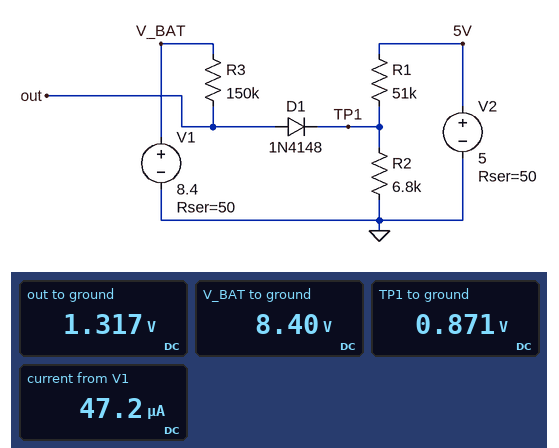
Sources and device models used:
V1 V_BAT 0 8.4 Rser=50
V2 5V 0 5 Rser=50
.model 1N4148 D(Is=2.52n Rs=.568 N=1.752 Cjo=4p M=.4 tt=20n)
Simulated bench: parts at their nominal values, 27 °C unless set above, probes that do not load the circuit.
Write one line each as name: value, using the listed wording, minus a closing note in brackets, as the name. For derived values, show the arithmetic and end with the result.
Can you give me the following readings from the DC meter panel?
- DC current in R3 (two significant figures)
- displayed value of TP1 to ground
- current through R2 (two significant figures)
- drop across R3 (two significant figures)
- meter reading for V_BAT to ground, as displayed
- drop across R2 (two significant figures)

DC current in R3: (8.4 V - 1.317 V) / 150 kΩ = 47 µA
displayed value of TP1 to ground: 0.871 V
current through R2: (871 mV) / 6.8 kΩ = 130 µA
drop across R3: 8.4 V - 1.317 V = 7.1 V
meter reading for V_BAT to ground, as displayed: 8.40 V
drop across R2: 871 mV = 870 mV
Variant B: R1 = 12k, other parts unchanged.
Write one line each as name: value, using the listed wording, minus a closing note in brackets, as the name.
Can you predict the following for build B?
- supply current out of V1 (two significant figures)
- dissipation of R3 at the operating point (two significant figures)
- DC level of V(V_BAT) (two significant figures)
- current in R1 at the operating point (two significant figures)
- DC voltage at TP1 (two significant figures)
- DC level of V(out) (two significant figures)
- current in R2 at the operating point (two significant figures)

supply current out of V1: 40 µA
dissipation of R3 at the operating point: 240 µW
DC level of V(V_BAT): 8.4 V
current in R1 at the operating point: 250 µA
DC voltage at TP1: 2.0 V
DC level of V(out): 2.4 V
current in R2 at the operating point: 290 µA
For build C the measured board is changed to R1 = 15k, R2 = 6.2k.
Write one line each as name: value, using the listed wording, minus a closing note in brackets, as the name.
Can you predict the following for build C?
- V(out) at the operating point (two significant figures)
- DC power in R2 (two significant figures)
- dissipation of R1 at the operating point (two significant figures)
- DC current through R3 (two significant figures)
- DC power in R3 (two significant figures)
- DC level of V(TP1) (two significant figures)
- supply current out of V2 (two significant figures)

V(out) at the operating point: 2.1 V
DC power in R2: 440 µW
dissipation of R1 at the operating point: 750 µW
DC current through R3: 42 µA
DC power in R3: 270 µW
DC level of V(TP1): 1.6 V
supply current out of V2: 220 µA
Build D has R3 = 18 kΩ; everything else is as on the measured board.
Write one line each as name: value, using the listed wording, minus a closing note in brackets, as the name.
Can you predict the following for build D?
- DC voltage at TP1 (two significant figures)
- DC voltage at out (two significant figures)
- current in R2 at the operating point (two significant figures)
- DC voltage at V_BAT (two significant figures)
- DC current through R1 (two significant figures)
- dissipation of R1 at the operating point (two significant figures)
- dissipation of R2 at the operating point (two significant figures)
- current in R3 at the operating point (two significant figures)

DC voltage at TP1: 2.4 V
DC voltage at out: 2.9 V
current in R2 at the operating point: 350 µA
DC voltage at V_BAT: 8.4 V
DC current through R1: 51 µA
dissipation of R1 at the operating point: 130 µW
dissipation of R2 at the operating point: 850 µW
current in R3 at the operating point: 300 µA
